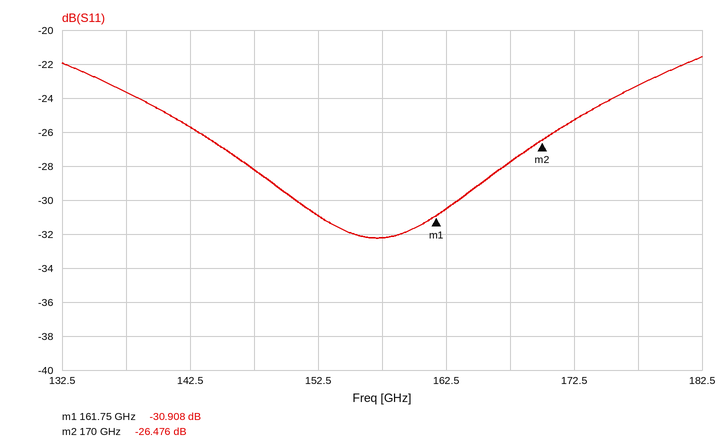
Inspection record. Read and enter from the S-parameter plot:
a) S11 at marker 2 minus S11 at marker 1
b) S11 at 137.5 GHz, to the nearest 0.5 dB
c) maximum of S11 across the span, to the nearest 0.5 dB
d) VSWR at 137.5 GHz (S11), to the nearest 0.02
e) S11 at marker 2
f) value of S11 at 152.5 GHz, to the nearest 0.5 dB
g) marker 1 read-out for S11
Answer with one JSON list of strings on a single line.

["4.432 dB", "-23.5 dB", "-21.5 dB", "1.14", "-26.476 dB", "-31.0 dB", "-30.908 dB"]
